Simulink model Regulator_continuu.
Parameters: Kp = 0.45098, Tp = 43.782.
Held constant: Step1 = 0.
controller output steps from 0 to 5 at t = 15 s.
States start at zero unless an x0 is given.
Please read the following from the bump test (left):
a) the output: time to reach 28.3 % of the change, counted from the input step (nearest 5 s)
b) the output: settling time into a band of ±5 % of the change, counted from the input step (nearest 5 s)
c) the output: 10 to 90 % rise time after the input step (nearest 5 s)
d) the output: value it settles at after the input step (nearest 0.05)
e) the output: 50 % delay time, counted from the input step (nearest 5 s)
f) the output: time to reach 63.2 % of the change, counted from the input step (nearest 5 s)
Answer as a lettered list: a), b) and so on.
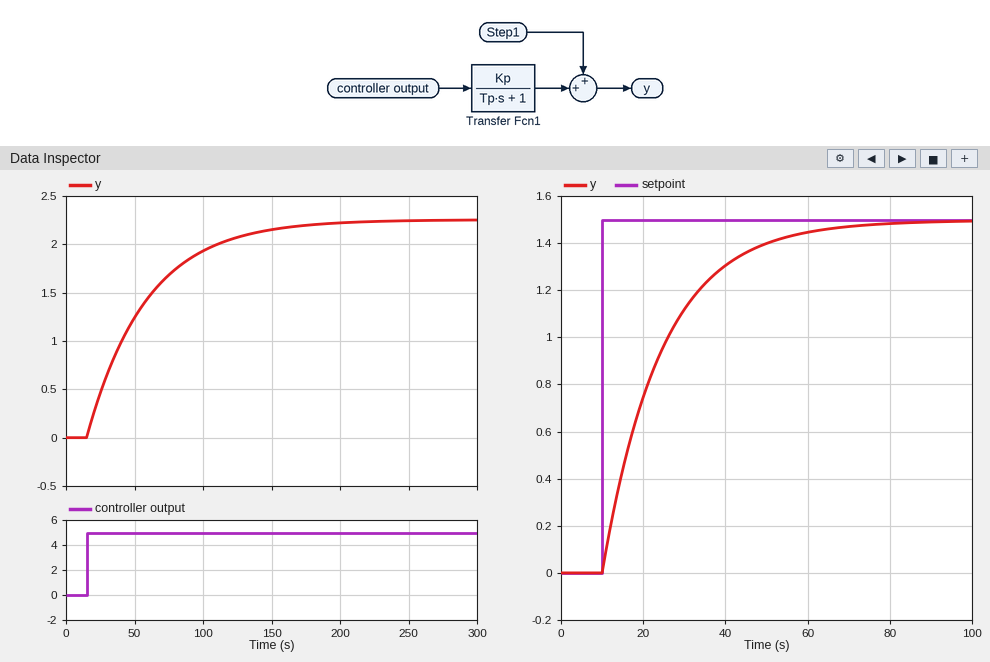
a) 15 s
b) 130 s
c) 95 s
d) 2.25
e) 30 s
f) 45 s
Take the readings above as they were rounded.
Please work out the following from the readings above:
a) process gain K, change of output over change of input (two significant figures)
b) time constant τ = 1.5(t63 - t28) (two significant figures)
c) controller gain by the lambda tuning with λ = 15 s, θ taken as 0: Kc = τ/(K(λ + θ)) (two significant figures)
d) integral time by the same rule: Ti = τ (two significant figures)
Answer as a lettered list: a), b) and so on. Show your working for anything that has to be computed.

a) (2.25 - 0) / 5 = 0.45
b) 1.5 × (45 - 15) = 45 s
c) 45 / (0.45 × (15 + 0)) = 6.7
d) 45 s
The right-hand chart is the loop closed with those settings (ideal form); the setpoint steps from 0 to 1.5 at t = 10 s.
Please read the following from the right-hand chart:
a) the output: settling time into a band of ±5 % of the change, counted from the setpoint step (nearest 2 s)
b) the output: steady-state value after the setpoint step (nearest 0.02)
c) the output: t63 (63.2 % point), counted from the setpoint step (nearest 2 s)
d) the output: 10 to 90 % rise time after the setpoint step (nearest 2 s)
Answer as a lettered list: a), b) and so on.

a) 44 s
b) 1.50
c) 14 s
d) 32 s
